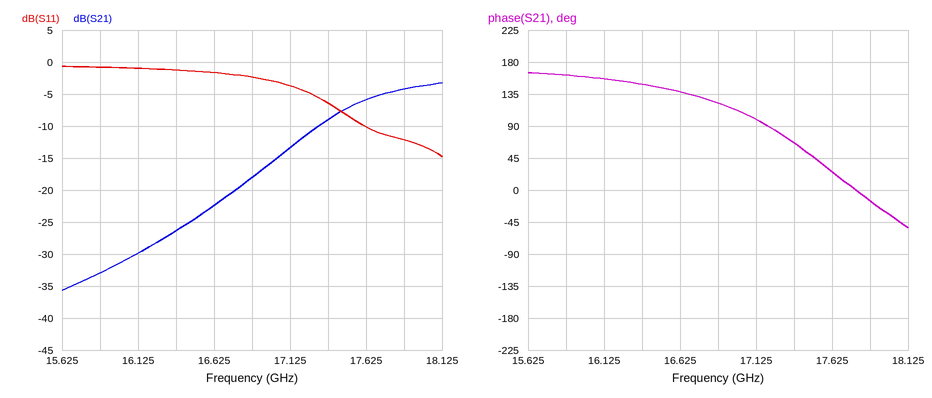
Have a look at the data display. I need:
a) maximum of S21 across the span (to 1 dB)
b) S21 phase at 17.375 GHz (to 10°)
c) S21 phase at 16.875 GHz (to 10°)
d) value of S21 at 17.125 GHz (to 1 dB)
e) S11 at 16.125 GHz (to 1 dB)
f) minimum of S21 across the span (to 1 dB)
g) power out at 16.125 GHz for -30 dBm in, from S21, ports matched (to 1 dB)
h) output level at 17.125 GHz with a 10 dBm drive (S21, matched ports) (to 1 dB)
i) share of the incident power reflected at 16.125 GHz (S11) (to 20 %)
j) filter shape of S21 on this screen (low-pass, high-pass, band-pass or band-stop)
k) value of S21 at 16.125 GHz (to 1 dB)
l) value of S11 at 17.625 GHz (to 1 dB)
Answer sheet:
-3 dB
70°
120°
-13 dB
-1 dB
-36 dB
-60 dBm
-3 dBm
80 %
high-pass
-30 dB
-10 dB
